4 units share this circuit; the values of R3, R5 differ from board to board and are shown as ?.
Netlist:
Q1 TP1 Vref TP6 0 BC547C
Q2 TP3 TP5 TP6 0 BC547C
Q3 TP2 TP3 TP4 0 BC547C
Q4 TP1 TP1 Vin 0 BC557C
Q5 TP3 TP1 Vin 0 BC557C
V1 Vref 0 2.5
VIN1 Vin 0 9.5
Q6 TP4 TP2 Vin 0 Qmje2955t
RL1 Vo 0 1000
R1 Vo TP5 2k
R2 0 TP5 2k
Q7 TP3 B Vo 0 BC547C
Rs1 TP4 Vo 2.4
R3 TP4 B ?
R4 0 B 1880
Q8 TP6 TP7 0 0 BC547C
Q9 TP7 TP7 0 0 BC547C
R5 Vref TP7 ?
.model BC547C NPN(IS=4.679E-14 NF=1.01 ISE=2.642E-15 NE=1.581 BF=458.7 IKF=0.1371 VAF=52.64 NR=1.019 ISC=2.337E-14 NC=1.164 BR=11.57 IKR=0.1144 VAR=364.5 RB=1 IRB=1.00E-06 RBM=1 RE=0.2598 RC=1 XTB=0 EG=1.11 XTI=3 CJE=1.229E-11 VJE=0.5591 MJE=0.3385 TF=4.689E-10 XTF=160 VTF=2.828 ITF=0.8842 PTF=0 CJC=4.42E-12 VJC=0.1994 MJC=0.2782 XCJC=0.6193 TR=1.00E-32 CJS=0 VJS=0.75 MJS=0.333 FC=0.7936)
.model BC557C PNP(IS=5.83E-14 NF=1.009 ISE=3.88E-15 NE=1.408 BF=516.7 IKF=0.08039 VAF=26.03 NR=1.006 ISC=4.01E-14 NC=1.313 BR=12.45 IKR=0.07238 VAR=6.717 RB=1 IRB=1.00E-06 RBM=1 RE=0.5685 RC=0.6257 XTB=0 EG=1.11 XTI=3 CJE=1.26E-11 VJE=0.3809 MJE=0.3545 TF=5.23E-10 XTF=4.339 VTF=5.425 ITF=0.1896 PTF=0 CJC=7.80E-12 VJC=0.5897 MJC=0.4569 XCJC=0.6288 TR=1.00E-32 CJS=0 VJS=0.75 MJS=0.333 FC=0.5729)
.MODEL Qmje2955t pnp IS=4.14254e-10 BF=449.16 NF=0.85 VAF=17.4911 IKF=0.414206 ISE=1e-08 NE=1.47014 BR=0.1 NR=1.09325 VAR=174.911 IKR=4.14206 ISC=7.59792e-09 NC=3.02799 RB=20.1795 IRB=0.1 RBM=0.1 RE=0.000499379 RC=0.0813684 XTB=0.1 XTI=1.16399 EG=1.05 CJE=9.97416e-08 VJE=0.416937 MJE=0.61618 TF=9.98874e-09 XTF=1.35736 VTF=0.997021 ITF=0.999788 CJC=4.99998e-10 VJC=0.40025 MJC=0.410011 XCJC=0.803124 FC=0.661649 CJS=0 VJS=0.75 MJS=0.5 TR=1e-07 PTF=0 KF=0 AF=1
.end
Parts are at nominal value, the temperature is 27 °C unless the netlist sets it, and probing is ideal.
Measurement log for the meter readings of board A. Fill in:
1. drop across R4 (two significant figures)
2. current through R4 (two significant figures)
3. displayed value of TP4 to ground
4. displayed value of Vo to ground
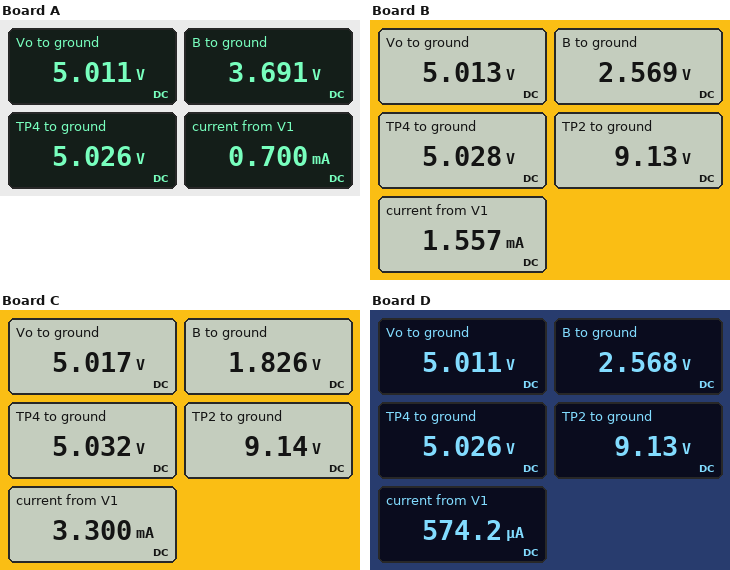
3.7 V
2.0 mA
5.026 V
5.011 V
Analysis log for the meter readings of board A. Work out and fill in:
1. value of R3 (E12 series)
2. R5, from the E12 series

680 Ω
2.7 kΩ
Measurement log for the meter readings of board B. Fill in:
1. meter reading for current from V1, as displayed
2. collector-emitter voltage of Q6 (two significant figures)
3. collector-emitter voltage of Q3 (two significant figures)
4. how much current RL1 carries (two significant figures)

1.557 mA
-4.5 V
4.1 V
5.0 mA
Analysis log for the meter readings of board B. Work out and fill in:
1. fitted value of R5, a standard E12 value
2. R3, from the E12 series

1.2 kΩ
1.8 kΩ
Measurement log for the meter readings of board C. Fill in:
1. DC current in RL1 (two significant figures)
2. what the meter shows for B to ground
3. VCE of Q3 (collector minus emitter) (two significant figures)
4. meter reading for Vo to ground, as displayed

5.0 mA
1.826 V
4.1 V
5.017 V
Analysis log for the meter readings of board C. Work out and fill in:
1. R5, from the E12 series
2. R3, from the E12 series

560 Ω
3.3 kΩ
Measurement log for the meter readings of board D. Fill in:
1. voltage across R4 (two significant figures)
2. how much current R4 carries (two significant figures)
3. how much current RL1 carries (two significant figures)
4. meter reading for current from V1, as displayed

2.6 V
1.4 mA
5.0 mA
574.2 µA
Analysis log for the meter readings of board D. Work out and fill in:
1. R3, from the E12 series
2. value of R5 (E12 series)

1.8 kΩ
3.3 kΩ
